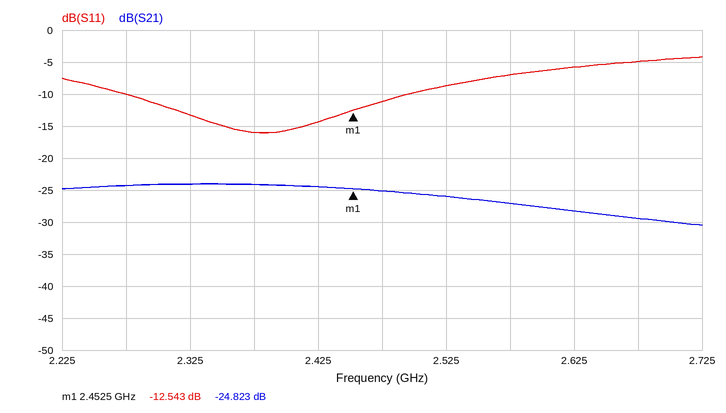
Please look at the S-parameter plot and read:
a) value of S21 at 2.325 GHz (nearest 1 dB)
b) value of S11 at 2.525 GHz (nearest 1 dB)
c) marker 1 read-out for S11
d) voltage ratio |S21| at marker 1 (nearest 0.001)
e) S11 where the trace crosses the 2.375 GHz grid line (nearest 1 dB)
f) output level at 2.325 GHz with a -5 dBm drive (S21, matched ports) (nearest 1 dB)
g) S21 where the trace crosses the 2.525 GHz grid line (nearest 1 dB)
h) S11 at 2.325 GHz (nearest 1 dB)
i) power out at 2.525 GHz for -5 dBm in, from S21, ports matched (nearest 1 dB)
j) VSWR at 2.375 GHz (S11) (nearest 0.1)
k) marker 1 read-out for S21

-24 dB
-9 dB
-12.543 dB
0.057
-16 dB
-29 dBm
-26 dB
-13 dB
-31 dBm
1.4
-24.823 dB
